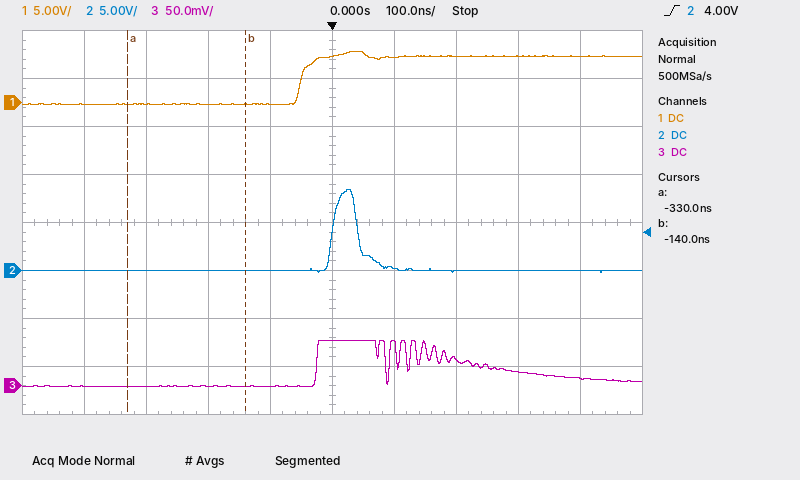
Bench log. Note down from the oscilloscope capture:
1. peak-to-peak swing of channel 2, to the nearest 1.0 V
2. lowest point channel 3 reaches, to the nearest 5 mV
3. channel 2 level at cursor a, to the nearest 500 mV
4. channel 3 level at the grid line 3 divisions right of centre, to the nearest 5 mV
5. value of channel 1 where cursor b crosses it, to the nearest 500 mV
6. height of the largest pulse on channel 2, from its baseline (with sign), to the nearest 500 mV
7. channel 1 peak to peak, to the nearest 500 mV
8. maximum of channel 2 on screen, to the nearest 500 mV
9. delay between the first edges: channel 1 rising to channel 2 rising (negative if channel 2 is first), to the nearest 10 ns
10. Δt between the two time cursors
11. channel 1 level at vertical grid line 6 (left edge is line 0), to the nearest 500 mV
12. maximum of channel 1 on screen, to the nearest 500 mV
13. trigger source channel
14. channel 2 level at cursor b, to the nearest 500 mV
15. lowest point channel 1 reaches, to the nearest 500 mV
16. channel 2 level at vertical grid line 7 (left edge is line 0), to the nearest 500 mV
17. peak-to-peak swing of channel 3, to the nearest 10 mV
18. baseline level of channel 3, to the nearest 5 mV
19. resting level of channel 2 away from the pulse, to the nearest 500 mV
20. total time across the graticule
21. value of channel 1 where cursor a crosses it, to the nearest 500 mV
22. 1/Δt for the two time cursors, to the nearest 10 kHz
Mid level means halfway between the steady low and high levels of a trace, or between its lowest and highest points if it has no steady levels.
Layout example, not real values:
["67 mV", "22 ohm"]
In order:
["9.0 V", "0 mV", "0.0 V", "15 mV", "0.0 V", "+8.5 V", "5.5 V", "8.5 V", "+50 ns", "190 ns", "4.5 V", "5.5 V", "channel 2", "0.0 V", "0.0 V", "0.0 V", "50 mV", "0 mV", "0.0 V", "1 µs", "0.0 V", "5.26 MHz"]
